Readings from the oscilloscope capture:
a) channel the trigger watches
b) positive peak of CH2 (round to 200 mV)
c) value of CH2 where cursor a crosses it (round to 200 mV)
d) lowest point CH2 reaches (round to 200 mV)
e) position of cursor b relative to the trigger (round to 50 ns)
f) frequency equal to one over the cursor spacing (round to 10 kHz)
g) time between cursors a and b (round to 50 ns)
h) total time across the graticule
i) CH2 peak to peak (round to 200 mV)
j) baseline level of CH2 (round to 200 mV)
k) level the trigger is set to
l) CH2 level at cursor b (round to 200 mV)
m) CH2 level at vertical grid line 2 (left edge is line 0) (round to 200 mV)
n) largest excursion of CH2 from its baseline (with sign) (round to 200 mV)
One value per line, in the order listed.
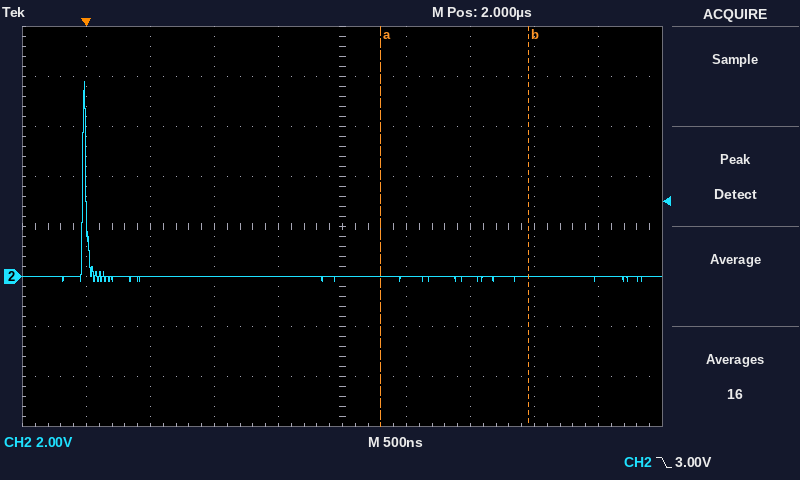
CH2
7.8 V
0.0 V
-200 mV
+3.45 µs
870 kHz
1.15 µs
5 µs
8.0 V
0.0 V
3.00 V
0.0 V
0.0 V
+7.8 V
